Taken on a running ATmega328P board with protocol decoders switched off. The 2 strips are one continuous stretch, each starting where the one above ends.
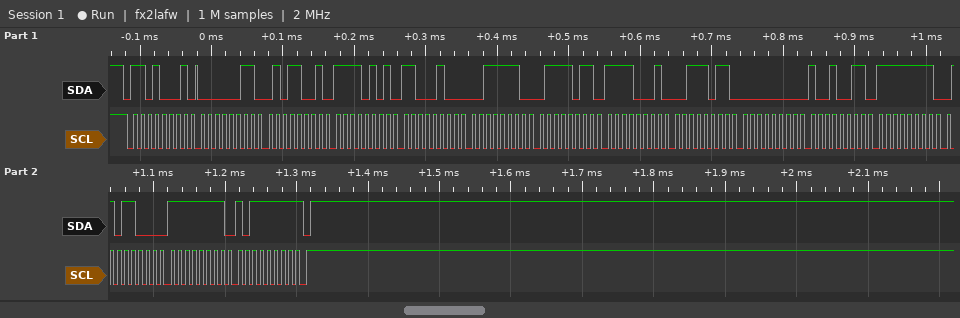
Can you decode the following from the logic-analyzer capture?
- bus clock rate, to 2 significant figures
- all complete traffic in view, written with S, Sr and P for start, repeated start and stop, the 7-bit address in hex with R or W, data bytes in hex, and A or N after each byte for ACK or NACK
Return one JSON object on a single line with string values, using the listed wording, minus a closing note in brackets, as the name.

{"bus clock rate, to 2 significant figures": "100 kHz", "all complete traffic in view, written with S, Sr and P for start, repeated start and stop, the 7-bit address in hex with R or W, data bytes in hex, and A or N after each byte for ACK or NACK": "S 68R A 03 A 59 A F5 A C4 A 3E A 7B A F1 A 3B A 00 A 93 A FF A 58 A FF A BF N P"}
